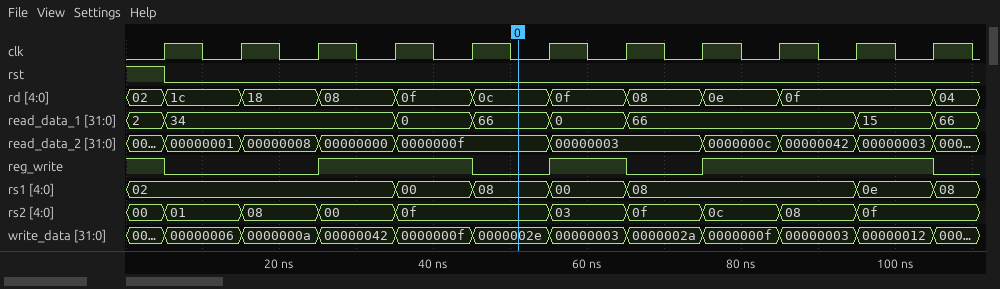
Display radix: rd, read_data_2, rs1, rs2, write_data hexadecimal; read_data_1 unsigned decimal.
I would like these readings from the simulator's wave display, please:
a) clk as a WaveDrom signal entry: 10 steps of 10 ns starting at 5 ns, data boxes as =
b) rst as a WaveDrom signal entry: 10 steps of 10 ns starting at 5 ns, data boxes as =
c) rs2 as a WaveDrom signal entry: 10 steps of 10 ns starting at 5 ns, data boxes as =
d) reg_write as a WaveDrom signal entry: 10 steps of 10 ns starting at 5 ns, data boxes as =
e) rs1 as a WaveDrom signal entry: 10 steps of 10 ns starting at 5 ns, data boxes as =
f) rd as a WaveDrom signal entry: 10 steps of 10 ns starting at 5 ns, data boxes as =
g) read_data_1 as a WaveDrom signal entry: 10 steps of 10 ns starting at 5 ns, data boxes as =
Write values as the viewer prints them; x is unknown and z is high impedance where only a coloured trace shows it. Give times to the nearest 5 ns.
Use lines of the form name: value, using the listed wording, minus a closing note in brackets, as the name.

clk as a WaveDrom signal entry: 10 steps of 10 ns starting at 5 ns, data boxes as =: {name: 'clk', wave: 'p.........'}
rst as a WaveDrom signal entry: 10 steps of 10 ns starting at 5 ns, data boxes as =: {name: 'rst', wave: '0.........'}
rs2 as a WaveDrom signal entry: 10 steps of 10 ns starting at 5 ns, data boxes as =: {name: 'rs2', wave: '====.=====', data: '01 08 00 0f 03 0f 0c 08 0f'}
reg_write as a WaveDrom signal entry: 10 steps of 10 ns starting at 5 ns, data boxes as =: {name: 'reg_write', wave: '0.1.0101..'}
rs1 as a WaveDrom signal entry: 10 steps of 10 ns starting at 5 ns, data boxes as =: {name: 'rs1', wave: '=..====..=', data: '02 00 08 00 08 0e'}
rd as a WaveDrom signal entry: 10 steps of 10 ns starting at 5 ns, data boxes as =: {name: 'rd', wave: '=========.', data: '1c 18 08 0f 0c 0f 08 0e 0f'}
read_data_1 as a WaveDrom signal entry: 10 steps of 10 ns starting at 5 ns, data boxes as =: {name: 'read_data_1', wave: '=..====..=', data: '34 0 66 0 66 15'}
